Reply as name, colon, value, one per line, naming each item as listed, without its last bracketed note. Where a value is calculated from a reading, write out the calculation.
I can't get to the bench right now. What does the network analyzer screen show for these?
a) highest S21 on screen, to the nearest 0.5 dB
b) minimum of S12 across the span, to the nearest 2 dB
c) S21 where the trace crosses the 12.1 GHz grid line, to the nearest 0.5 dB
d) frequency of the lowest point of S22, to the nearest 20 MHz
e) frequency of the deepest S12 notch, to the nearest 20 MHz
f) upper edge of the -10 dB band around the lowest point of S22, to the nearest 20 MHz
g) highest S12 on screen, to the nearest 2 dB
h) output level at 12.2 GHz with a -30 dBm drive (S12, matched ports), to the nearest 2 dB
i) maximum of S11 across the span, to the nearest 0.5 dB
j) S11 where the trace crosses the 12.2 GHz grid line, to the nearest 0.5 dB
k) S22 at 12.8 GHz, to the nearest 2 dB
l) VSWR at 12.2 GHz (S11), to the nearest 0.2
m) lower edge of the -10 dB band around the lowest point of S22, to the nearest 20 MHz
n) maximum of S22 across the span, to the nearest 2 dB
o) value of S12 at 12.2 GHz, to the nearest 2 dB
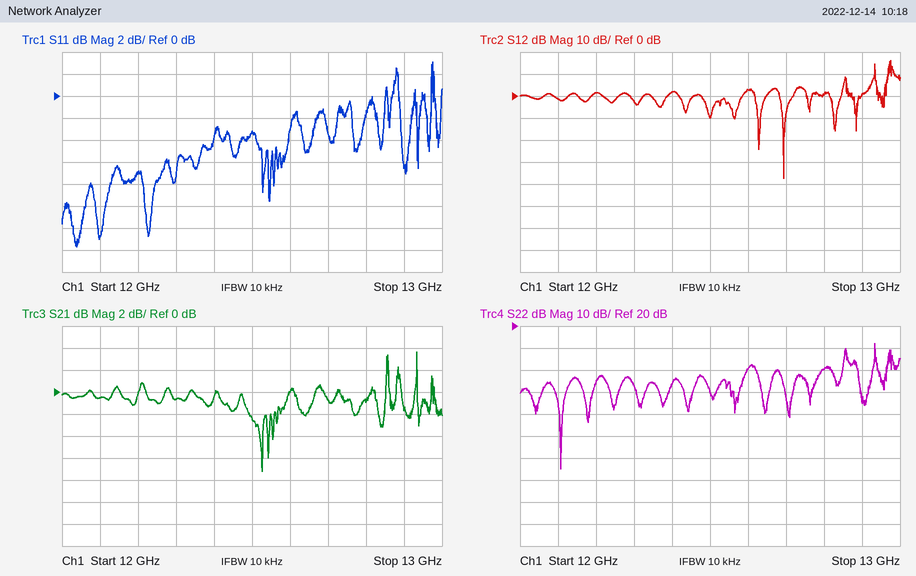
highest S21 on screen, to the nearest 0.5 dB: 3.5 dB
minimum of S12 across the span, to the nearest 2 dB: -38 dB
S21 where the trace crosses the 12.1 GHz grid line, to the nearest 0.5 dB: -0.5 dB
frequency of the lowest point of S22, to the nearest 20 MHz: 12.10 GHz
frequency of the deepest S12 notch, to the nearest 20 MHz: 12.70 GHz
upper edge of the -10 dB band around the lowest point of S22, to the nearest 20 MHz: 12.12 GHz
highest S12 on screen, to the nearest 2 dB: 16 dB
output level at 12.2 GHz with a -30 dBm drive (S12, matched ports), to the nearest 2 dB: -30 dBm + (2 dB) = -28 dBm
maximum of S11 across the span, to the nearest 0.5 dB: 3.0 dB
S11 where the trace crosses the 12.2 GHz grid line, to the nearest 0.5 dB: -7.0 dB
S22 at 12.8 GHz, to the nearest 2 dB: 0 dB
VSWR at 12.2 GHz (S11), to the nearest 0.2: |Γ| = 10^(-7/20) = 0.4467; VSWR = (1 + 0.4467)/(1 − 0.4467) ≈ 2.6
lower edge of the -10 dB band around the lowest point of S22, to the nearest 20 MHz: 12.10 GHz
maximum of S22 across the span, to the nearest 2 dB: 12 dB
value of S12 at 12.2 GHz, to the nearest 2 dB: 2 dB
